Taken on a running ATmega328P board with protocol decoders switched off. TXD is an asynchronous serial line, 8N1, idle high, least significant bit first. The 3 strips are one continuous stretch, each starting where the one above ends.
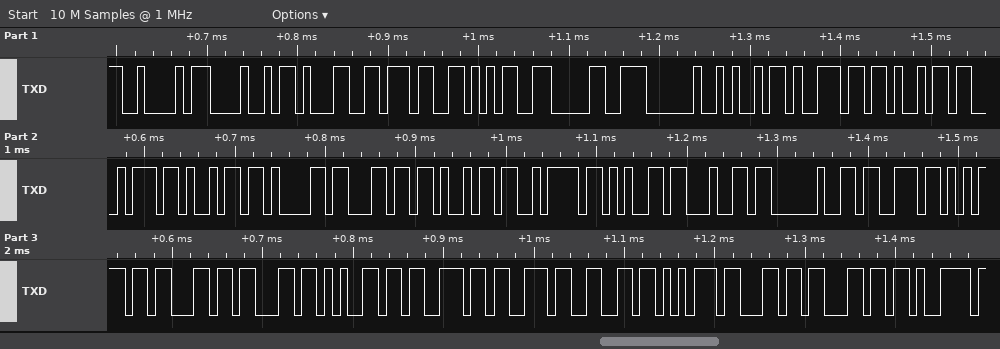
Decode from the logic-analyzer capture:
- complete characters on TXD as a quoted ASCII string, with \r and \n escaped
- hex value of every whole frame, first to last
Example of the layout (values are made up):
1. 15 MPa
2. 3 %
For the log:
1. "BH1750 initialized successfully"
2. 0x42 0x48 0x31 0x37 0x35 0x30 0x20 0x69 0x6E 0x69 0x74 0x69 0x61 0x6C 0x69 0x7A 0x65 0x64 0x20 0x73 0x75 0x63 0x63 0x65 0x73 0x73 0x66 0x75 0x6C 0x6C 0x79
